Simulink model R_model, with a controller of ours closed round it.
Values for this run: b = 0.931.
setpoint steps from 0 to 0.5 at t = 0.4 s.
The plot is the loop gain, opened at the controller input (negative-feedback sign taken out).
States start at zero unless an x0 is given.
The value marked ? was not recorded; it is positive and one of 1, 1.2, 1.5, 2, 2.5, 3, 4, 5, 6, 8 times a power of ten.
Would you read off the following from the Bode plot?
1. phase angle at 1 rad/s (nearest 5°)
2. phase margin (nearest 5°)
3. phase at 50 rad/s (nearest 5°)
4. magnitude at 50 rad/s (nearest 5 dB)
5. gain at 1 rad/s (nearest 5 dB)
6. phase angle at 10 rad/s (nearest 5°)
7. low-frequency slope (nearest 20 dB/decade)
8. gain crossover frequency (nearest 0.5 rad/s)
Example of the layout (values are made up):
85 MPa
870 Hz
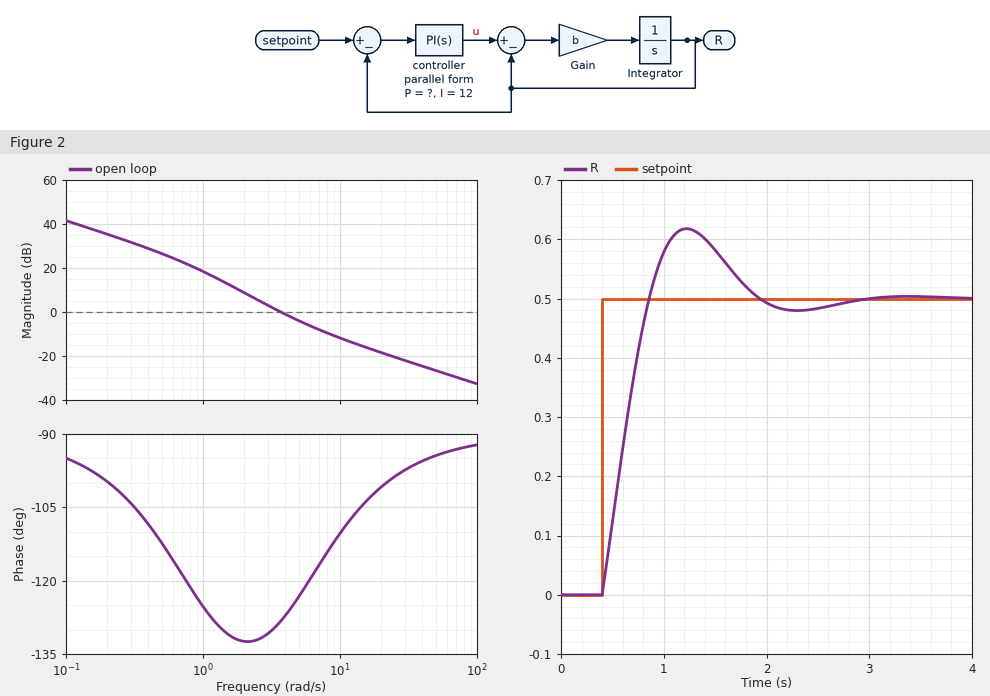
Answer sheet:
-125°
50°
-95°
-25 dB
20 dB
-110°
-20 dB/decade
3.5 rad/s
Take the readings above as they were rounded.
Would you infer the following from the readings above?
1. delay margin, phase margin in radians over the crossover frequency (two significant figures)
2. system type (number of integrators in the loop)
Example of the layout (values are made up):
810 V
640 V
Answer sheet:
0.25 s
1
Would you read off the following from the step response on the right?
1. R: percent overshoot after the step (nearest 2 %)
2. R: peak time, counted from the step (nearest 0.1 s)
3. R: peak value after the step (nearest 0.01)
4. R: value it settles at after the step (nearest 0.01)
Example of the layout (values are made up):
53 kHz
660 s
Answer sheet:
24 %
0.8 s
0.62
0.50
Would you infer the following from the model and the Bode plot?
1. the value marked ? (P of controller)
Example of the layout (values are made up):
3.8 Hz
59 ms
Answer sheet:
2.5
